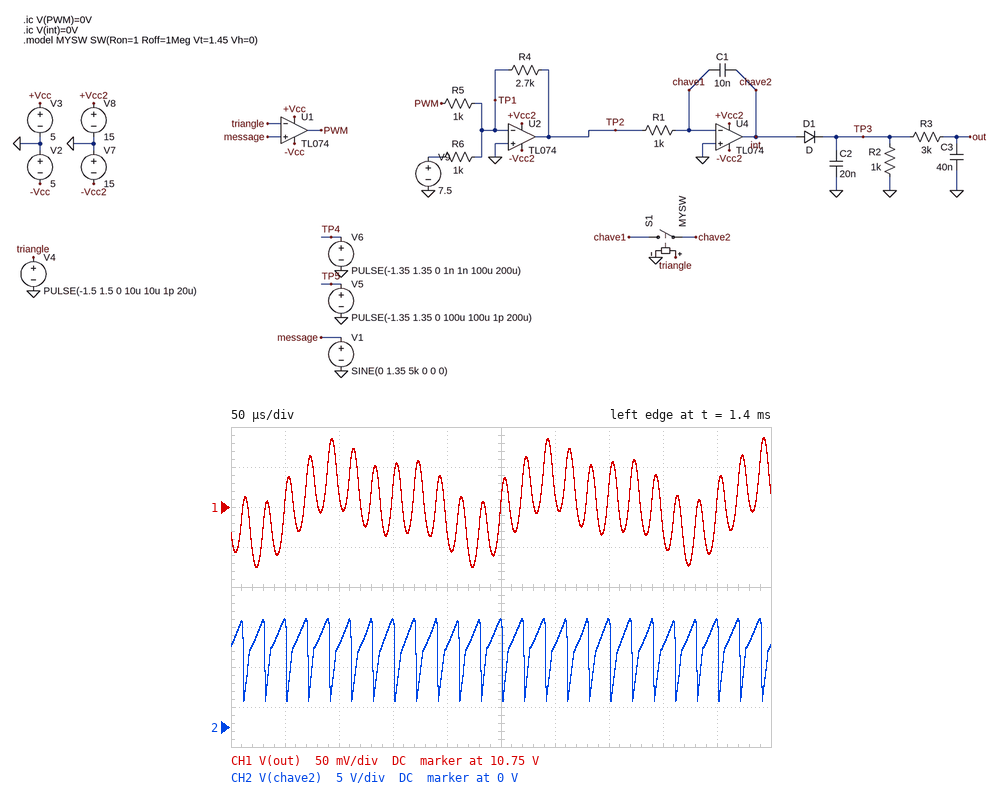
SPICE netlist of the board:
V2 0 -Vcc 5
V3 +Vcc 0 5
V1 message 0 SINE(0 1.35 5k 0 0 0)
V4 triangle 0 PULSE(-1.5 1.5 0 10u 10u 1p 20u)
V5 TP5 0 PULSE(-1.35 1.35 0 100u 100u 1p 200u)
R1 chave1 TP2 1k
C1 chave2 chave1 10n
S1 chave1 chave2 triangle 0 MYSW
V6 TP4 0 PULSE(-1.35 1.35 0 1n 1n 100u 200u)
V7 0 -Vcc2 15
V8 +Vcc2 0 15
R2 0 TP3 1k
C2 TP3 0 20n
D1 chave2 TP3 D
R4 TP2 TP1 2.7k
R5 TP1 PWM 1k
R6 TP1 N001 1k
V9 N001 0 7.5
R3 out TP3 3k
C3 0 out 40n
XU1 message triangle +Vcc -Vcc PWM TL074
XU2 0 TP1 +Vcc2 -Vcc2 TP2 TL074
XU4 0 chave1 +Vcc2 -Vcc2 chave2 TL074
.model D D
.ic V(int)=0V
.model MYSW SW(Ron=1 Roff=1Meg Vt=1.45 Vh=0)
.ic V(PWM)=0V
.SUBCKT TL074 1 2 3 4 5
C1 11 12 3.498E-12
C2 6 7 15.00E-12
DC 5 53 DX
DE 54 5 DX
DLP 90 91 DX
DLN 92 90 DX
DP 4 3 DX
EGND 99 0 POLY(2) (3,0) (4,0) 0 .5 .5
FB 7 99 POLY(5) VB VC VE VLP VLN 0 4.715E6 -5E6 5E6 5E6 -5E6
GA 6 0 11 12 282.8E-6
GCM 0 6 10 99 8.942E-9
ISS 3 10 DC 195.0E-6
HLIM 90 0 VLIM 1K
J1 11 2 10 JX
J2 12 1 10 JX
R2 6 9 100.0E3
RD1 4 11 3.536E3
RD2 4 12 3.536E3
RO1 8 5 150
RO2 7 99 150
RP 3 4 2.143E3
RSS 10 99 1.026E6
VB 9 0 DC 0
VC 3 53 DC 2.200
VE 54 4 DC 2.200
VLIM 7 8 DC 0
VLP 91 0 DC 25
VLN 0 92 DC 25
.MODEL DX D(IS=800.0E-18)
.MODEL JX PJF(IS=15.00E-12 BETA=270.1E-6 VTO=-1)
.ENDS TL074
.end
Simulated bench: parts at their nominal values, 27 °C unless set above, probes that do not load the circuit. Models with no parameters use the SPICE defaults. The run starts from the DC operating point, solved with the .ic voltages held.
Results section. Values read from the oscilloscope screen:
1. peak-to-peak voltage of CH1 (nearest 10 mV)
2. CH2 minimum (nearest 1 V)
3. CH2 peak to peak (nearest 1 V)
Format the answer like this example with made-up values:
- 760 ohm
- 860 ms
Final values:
- 160 mV
- 3 V
- 10 V
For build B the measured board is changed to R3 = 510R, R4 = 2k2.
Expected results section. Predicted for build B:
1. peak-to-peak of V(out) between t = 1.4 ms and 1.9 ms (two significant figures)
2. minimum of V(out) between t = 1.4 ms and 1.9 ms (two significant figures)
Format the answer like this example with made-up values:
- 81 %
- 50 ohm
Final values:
- 1.0 V
- 10 V
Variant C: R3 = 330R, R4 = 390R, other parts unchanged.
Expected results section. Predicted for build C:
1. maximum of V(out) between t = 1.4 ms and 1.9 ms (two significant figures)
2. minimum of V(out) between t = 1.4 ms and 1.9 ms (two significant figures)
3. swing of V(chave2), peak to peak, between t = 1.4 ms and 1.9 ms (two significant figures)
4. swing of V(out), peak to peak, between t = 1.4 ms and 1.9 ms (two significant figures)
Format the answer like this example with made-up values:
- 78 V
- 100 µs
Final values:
- 5.9 V
- 2.1 V
- 8.5 V
- 3.8 V
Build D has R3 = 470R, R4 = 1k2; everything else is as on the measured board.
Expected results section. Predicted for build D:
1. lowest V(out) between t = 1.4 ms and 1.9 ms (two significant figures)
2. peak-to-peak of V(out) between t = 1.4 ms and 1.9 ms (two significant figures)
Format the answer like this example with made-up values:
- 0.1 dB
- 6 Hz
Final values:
- 7.5 V
- 3.0 V
